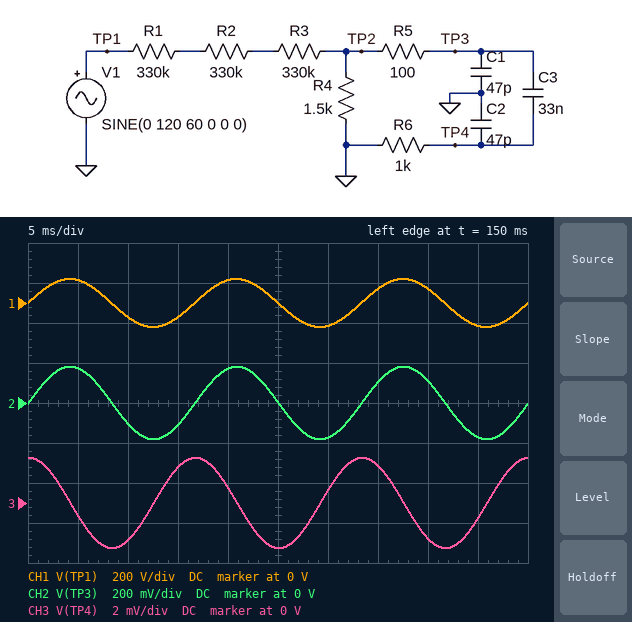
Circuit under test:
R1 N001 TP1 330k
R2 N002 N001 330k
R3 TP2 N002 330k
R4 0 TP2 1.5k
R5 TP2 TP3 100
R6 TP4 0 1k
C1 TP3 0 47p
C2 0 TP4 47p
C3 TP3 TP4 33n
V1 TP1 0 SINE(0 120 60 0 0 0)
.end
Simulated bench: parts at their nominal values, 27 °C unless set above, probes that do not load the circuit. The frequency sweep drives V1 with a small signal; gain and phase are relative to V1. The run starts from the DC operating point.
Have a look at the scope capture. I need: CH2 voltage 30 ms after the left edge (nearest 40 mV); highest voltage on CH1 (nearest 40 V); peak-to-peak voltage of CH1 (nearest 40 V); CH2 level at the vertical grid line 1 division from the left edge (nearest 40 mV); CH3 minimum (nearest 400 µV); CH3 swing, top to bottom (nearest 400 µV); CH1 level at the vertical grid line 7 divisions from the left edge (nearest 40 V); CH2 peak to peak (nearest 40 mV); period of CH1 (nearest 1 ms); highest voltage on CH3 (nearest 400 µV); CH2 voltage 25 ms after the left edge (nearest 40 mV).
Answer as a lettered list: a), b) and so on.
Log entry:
a) -160 mV
b) 120 V
c) 240 V
d) 160 mV
e) -2.4 mV
f) 4.4 mV
g) 80 V
h) 360 mV
i) 17 ms
j) 2.4 mV
k) 0 V
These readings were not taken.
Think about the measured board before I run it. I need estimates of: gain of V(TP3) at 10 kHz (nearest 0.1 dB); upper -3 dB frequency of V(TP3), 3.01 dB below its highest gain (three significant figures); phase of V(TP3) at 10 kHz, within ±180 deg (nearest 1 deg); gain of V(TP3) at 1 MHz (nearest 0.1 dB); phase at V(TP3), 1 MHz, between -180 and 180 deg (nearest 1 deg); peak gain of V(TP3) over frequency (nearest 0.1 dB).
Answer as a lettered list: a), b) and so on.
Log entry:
a) -63.9 dB
b) 2.21 kHz
c) -15 deg
d) -65.2 dB
e) -20 deg
f) -56.4 dB
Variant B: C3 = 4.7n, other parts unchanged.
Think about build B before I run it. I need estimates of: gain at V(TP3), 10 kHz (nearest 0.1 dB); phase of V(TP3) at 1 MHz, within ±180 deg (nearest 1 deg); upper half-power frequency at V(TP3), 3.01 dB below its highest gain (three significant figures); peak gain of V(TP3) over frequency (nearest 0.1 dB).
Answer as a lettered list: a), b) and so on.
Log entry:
a) -58.1 dB
b) -21 deg
c) 15.5 kHz
d) -56.4 dB
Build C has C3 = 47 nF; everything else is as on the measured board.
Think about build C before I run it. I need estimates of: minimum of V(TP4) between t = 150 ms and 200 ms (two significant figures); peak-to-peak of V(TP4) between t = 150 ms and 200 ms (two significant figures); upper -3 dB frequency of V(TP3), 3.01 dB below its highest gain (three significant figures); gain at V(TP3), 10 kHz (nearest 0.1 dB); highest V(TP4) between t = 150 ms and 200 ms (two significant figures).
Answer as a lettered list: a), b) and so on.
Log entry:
a) -3.2 mV
b) 6.4 mV
c) 1.55 kHz
d) -64.3 dB
e) 3.2 mV
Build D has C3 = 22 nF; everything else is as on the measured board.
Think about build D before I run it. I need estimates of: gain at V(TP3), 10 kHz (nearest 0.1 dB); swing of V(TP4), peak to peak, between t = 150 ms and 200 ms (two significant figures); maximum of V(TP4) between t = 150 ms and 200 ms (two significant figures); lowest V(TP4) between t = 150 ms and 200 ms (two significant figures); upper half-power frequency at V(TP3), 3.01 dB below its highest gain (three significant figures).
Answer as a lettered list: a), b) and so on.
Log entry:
a) -63.2 dB
b) 3.0 mV
c) 1.5 mV
d) -1.5 mV
e) 3.32 kHz
